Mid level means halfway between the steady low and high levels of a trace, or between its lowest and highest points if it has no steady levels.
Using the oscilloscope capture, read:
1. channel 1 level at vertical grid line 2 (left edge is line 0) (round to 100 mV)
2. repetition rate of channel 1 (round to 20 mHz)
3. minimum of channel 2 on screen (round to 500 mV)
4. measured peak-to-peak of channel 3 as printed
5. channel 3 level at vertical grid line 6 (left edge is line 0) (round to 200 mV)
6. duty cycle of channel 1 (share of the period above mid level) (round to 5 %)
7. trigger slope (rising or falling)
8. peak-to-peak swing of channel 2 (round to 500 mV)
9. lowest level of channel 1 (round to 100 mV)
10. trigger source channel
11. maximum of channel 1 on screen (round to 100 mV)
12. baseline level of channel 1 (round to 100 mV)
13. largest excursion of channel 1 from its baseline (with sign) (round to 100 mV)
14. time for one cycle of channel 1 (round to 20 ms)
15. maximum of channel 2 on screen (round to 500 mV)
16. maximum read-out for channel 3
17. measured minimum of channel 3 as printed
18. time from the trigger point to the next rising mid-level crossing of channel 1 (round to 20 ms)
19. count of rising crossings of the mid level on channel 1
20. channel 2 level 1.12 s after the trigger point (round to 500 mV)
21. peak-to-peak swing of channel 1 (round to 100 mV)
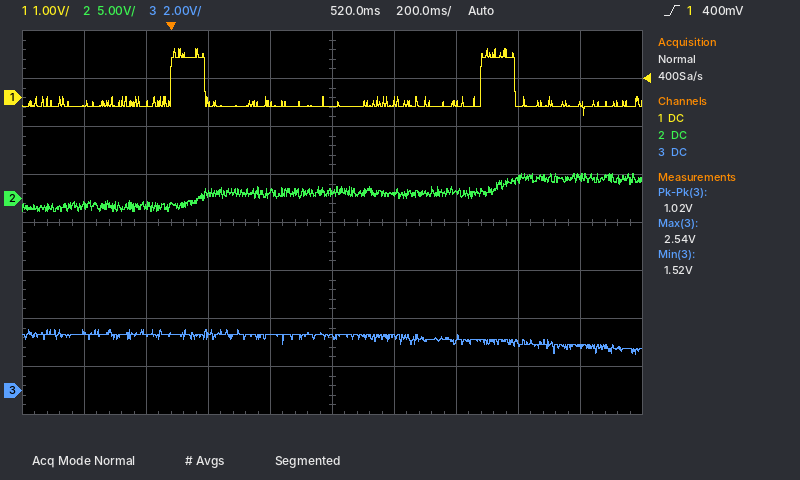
-100 mV
1.00 Hz
-1.5 V
1.02 V
2.2 V
10 %
rising
4.0 V
-400 mV
channel 1
1.0 V
-200 mV
+1.2 V
1.00 s
2.5 V
2.54 V
1.52 V
1.00 s
2
2.0 V
1.4 V
